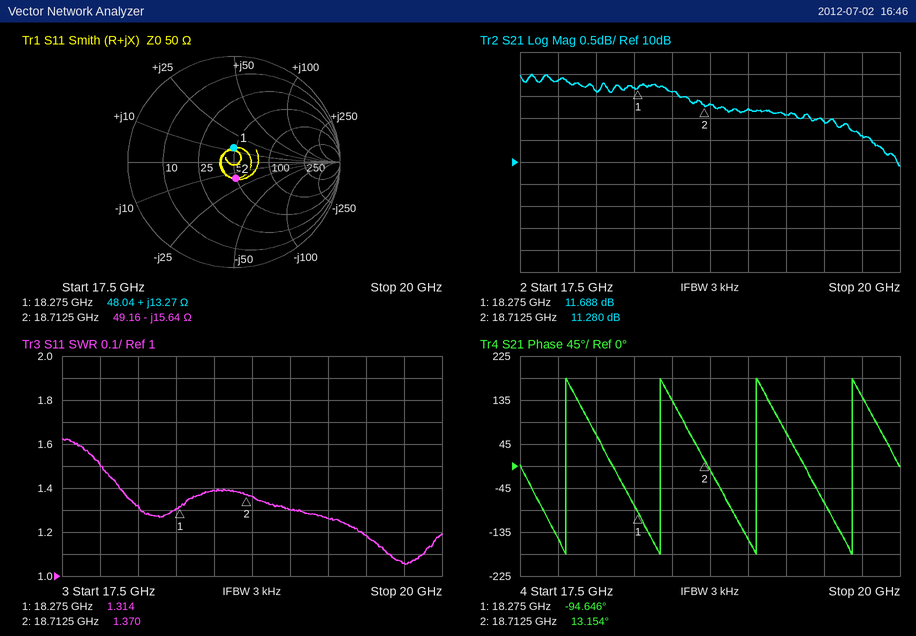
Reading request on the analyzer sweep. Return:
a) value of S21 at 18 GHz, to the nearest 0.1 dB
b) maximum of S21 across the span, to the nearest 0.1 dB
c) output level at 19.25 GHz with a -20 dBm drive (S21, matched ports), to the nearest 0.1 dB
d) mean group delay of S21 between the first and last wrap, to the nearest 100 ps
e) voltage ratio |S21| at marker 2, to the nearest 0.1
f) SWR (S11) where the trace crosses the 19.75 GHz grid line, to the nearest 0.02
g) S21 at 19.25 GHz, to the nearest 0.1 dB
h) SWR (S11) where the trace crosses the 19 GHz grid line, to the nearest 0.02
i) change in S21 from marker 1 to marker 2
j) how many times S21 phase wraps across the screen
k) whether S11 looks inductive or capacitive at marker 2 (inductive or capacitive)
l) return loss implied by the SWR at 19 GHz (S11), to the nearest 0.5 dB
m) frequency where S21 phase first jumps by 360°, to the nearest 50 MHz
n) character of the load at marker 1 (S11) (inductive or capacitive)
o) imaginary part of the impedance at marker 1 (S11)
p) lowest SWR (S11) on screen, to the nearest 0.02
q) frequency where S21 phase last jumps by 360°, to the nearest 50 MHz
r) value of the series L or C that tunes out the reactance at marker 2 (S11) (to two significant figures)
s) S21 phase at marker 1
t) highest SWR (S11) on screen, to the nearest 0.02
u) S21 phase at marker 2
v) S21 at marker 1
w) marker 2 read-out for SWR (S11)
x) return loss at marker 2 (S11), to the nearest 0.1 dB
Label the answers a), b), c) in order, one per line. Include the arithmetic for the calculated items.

a) 11.6 dB
b) 12.0 dB
c) -20 dBm + (11.1 dB) = -8.9 dBm
d) 3 cycles / (19.70 GHz − 17.80 GHz) ≈ 1.6 ns
e) 10^(11.28/20) ≈ 3.7
f) 1.06
g) 11.1 dB
h) 1.30
i) 11.28 − (11.688) = -0.408 dB
j) 4
k) capacitive
l) −20 log10((1.3 − 1)/(1.3 + 1)) ≈ 17.7 dB, so 17.5 dB to the nearest 0.5 dB
m) 17.80 GHz
n) inductive
o) +13.27 Ω
p) 1.06
q) 19.70 GHz
r) L = 15.64 Ω/(2π × 18.7125 GHz) ≈ 133 pH, so 130 pH to two significant figures
s) -94.646°
t) 1.62
u) 13.154°
v) 11.688 dB
w) 1.370
x) 16.1 dB
